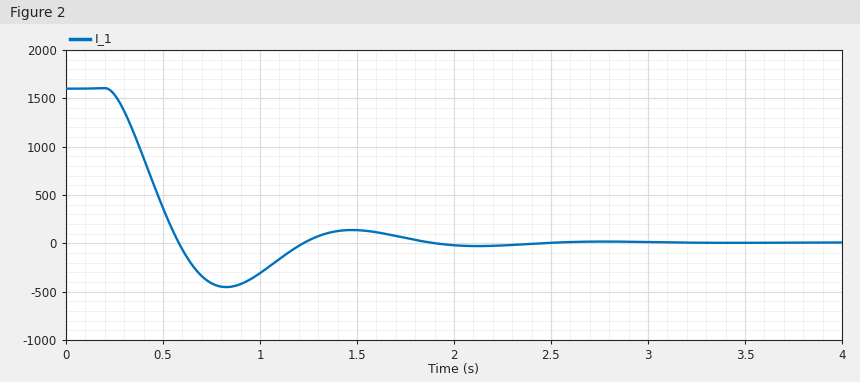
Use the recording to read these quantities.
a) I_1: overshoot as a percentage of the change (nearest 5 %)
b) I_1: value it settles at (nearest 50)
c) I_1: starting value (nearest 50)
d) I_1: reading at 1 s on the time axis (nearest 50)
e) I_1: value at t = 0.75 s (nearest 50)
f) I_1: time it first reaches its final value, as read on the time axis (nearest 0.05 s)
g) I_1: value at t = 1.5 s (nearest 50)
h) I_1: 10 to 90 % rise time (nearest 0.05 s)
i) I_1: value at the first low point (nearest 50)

30 %
0
1600
-300
-400
0.60 s
150
0.25 s
-450
